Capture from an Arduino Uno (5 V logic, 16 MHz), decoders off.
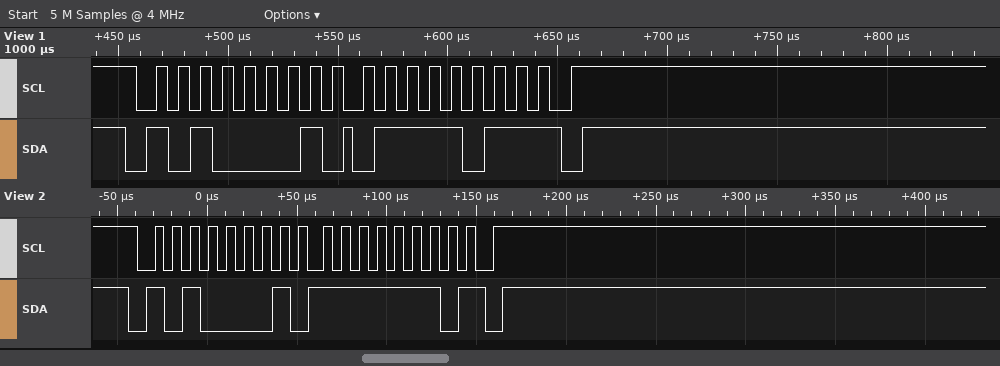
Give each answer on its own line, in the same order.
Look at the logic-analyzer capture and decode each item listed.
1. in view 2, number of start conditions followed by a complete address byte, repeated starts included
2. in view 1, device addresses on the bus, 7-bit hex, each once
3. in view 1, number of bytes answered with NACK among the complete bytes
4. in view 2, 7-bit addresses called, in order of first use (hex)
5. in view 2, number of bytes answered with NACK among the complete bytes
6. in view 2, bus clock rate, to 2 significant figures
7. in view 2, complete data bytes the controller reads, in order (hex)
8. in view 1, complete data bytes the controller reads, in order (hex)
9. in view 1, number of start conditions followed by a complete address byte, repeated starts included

1
0x50
1
0x50
1
100 kHz
FE
7B
1
